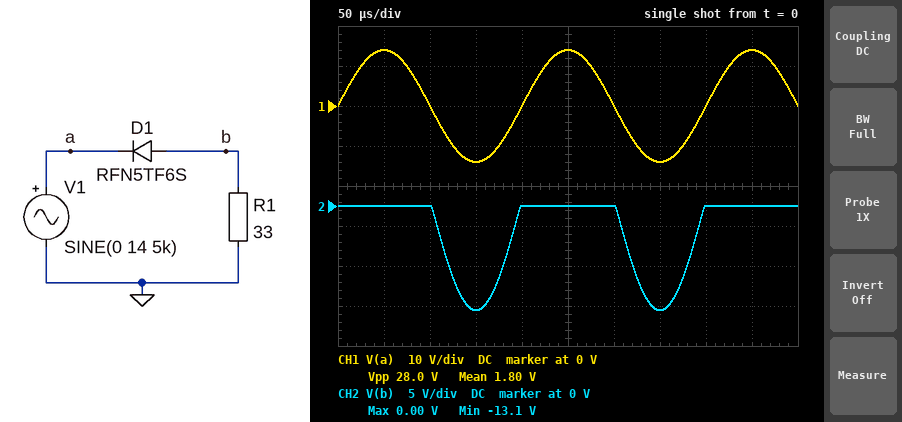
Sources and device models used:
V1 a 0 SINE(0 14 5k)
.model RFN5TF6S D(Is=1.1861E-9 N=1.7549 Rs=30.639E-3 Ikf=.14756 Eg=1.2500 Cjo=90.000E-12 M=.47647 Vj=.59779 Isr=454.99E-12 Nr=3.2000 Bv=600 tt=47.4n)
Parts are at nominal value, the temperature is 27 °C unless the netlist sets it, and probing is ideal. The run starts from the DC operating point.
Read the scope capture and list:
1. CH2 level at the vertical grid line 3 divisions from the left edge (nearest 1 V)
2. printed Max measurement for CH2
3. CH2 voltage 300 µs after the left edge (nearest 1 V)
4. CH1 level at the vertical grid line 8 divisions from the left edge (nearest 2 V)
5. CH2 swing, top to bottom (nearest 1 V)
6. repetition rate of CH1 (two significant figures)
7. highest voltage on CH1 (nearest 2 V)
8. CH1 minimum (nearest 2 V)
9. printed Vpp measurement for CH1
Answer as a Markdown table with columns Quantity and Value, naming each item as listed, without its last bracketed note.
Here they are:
| Quantity | Value |
|---|---|
| CH2 level at the vertical grid line 3 divisions from the left edge | -13 V |
| printed Max measurement for CH2 | 0.00 V |
| CH2 voltage 300 µs after the left edge | 0 V |
| CH1 level at the vertical grid line 8 divisions from the left edge | 0 V |
| CH2 swing, top to bottom | 13 V |
| repetition rate of CH1 | 5.0 kHz |
| highest voltage on CH1 | 14 V |
| CH1 minimum | -14 V |
| printed Vpp measurement for CH1 | 28.0 V |
